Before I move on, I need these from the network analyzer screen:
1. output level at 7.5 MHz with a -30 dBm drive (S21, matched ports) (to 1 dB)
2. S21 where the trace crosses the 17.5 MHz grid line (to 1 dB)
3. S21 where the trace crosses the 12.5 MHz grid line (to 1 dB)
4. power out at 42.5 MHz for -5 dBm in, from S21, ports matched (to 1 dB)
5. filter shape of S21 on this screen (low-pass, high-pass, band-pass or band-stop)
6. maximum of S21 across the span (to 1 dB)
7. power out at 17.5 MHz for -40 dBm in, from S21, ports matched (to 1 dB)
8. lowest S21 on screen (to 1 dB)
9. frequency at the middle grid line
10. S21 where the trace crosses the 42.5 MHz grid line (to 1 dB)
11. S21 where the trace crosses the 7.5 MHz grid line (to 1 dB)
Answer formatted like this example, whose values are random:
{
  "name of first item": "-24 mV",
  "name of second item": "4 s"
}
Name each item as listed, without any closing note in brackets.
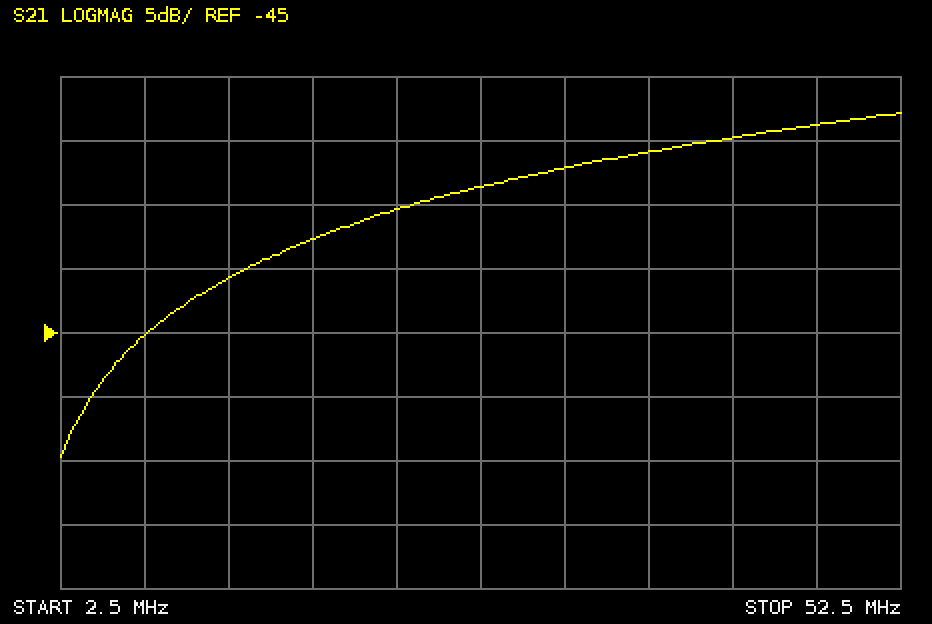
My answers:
{
  "output level at 7.5 MHz with a -30 dBm drive (S21, matched ports)": "-75 dBm",
  "S21 where the trace crosses the 17.5 MHz grid line": "-38 dB",
  "S21 where the trace crosses the 12.5 MHz grid line": "-41 dB",
  "power out at 42.5 MHz for -5 dBm in, from S21, ports matched": "-35 dBm",
  "filter shape of S21 on this screen": "high-pass",
  "maximum of S21 across the span": "-28 dB",
  "power out at 17.5 MHz for -40 dBm in, from S21, ports matched": "-78 dBm",
  "lowest S21 on screen": "-55 dB",
  "frequency at the middle grid line": "27.5 MHz",
  "S21 where the trace crosses the 42.5 MHz grid line": "-30 dB",
  "S21 where the trace crosses the 7.5 MHz grid line": "-45 dB"
}
